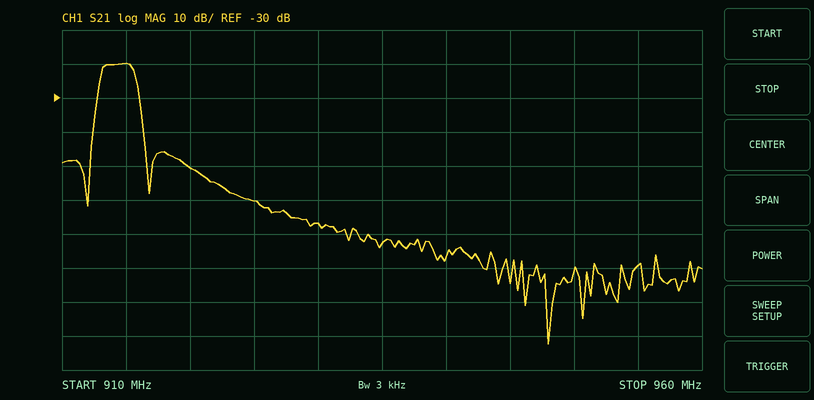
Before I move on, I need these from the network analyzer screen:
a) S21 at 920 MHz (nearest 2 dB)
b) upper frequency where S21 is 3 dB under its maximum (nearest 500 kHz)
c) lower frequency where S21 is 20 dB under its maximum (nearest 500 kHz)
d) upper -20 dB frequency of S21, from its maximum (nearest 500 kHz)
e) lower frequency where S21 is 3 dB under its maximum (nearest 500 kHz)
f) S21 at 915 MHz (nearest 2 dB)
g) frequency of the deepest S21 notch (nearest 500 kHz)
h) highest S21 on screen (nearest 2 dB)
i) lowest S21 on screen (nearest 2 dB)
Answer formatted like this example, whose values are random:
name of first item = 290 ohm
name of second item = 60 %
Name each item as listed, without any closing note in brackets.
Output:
S21 at 920 MHz = -50 dB
upper frequency where S21 is 3 dB under its maximum = 915.5 MHz
lower frequency where S21 is 20 dB under its maximum = 912.5 MHz
upper -20 dB frequency of S21, from its maximum = 916.5 MHz
lower frequency where S21 is 3 dB under its maximum = 913.0 MHz
S21 at 915 MHz = -20 dB
frequency of the deepest S21 notch = 948.0 MHz
highest S21 on screen = -20 dB
lowest S21 on screen = -102 dB
